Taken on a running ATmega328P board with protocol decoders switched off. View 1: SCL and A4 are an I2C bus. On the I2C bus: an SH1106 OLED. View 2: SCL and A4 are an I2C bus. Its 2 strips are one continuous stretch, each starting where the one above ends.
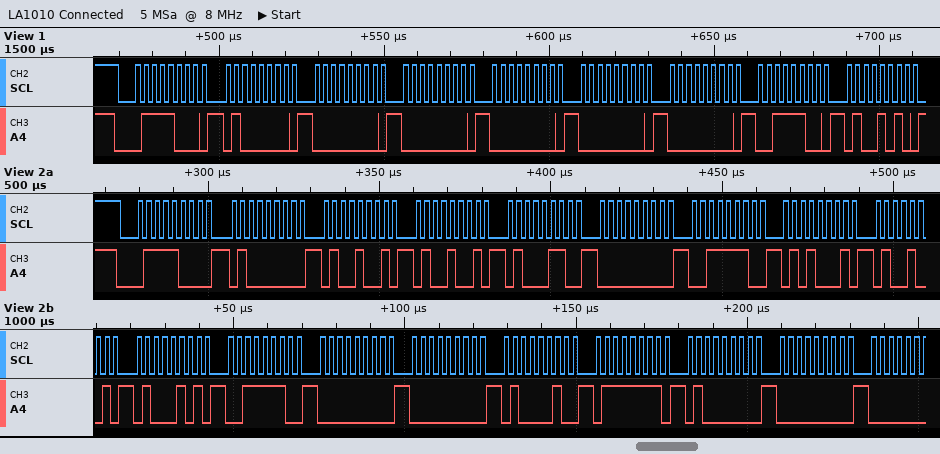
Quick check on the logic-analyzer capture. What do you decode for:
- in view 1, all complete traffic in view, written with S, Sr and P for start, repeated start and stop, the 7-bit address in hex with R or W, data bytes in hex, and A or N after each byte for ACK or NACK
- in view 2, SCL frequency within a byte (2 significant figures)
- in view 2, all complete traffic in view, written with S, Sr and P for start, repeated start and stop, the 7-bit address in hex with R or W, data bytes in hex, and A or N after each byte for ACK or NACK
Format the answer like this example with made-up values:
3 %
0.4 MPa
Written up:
S 3CW A 40 A 00 A 00 A 00 A 00 A 00 A 3C A 4A A
400 kHz
S 3CW A 40 A 49 A 49 A 46 A 00 A 3E A 51 A 49 A 45 A 3E A 00 A 00 A 42 A 7F A 40 A 00 A
